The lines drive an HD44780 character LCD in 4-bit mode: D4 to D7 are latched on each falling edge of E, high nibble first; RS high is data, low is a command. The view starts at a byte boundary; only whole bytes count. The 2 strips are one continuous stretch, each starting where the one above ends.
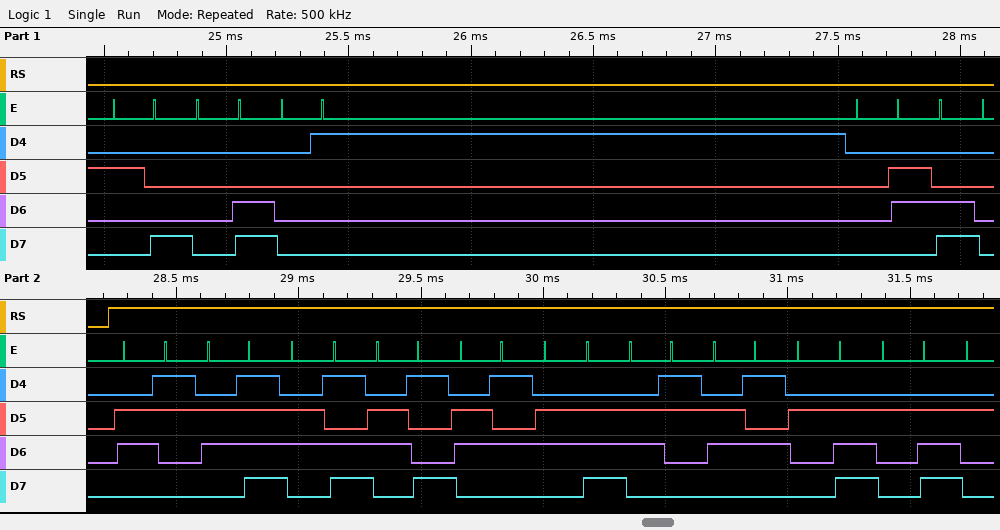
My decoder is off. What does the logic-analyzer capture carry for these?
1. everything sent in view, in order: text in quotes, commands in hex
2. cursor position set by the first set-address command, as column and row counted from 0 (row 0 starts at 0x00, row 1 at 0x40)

0x28 0x0C 0x01 0x06 0xC0 "comience.."
column 0, row 1
